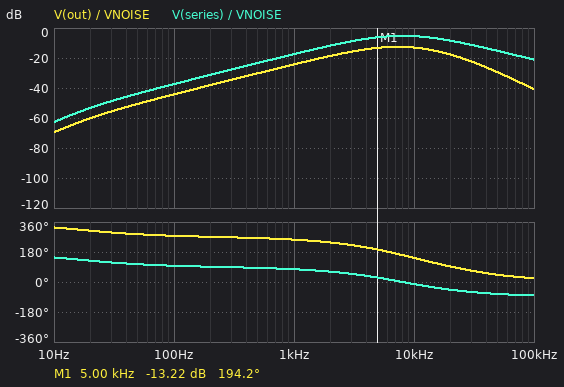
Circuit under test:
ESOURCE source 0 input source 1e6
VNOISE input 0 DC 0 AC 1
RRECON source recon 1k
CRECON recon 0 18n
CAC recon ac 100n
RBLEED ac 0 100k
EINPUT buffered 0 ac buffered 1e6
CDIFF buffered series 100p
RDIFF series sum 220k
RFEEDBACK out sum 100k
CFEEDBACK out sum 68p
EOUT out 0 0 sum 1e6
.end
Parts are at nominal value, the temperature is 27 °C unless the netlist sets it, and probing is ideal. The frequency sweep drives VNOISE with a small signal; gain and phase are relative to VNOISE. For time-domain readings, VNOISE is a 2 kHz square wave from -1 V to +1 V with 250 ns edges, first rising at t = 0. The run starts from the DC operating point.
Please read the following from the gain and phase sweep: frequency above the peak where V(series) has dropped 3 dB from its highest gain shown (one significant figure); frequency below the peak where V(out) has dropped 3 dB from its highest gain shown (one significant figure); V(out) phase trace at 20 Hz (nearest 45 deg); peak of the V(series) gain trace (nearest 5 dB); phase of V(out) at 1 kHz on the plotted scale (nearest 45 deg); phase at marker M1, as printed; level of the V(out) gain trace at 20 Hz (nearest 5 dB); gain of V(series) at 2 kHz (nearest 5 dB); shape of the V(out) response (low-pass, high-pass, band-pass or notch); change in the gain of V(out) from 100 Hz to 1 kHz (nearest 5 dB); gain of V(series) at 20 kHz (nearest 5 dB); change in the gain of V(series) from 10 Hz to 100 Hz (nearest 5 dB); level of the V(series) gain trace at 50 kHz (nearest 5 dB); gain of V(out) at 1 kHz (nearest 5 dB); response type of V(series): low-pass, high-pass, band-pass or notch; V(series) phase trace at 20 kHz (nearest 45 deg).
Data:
20 kHz
3 kHz
315 deg
-5 dB
270 deg
194.2 deg
-60 dB
-10 dB
band-pass
20 dB
-10 dB
25 dB
-15 dB
-25 dB
band-pass
-45 deg
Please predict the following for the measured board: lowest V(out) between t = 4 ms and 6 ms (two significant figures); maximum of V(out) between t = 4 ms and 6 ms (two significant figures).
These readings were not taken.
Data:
-340 mV
340 mV
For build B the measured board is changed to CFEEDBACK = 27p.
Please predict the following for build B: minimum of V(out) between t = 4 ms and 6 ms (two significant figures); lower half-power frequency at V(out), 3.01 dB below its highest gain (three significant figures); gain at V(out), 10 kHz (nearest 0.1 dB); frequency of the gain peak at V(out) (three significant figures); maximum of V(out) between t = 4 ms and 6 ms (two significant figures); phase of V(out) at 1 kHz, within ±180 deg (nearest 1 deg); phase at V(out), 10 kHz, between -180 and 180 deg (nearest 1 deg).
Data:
-360 mV
3.28 kHz
-12.4 dB
7.90 kHz
360 mV
-104 deg
158 deg
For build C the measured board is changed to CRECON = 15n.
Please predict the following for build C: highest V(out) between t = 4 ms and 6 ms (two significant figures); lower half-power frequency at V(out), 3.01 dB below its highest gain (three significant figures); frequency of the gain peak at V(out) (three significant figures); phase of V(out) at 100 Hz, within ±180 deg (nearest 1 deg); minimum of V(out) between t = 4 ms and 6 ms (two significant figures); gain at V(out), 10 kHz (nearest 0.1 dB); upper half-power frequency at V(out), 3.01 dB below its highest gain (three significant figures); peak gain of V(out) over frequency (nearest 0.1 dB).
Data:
370 mV
3.36 kHz
7.91 kHz
-83 deg
-370 mV
-12.2 dB
17.0 kHz
-11.9 dB
